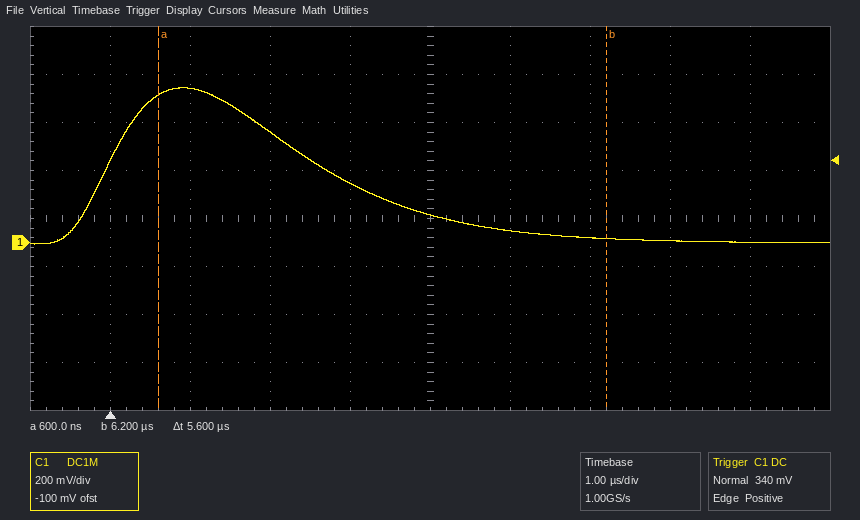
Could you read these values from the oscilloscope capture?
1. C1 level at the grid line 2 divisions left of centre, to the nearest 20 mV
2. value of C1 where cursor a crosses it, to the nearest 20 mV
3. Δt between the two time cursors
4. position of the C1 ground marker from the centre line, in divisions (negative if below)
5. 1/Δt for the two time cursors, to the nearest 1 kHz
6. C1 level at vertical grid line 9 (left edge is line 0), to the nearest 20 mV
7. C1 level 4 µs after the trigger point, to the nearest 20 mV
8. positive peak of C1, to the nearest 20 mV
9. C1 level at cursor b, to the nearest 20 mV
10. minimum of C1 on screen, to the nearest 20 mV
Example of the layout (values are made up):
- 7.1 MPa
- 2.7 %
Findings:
- 460 mV
- 620 mV
- 5.6 µs
- -0.5 div
- 179 kHz
- 0 mV
- 120 mV
- 640 mV
- 20 mV
- 0 mV
